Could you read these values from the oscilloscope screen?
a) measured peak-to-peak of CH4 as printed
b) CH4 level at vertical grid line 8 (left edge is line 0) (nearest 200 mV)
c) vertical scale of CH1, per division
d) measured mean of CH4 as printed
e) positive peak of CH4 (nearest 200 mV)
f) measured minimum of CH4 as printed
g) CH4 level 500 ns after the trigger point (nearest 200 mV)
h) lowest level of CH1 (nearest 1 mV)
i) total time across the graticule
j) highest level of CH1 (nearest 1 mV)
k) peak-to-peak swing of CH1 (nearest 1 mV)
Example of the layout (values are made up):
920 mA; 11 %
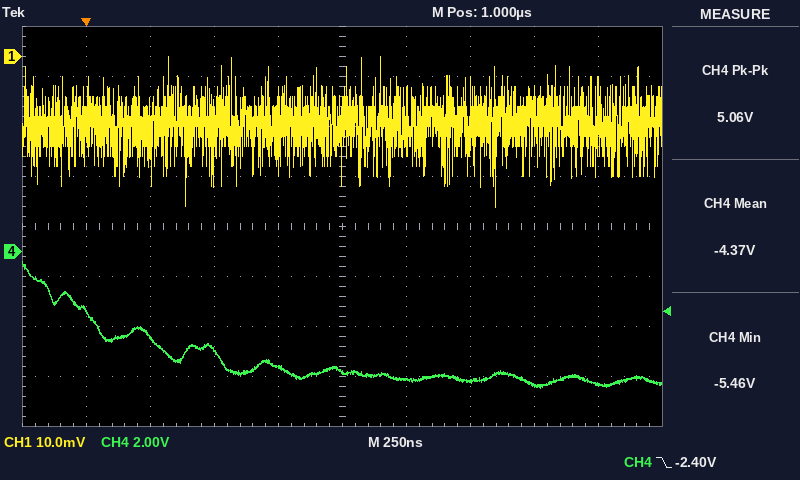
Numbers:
5.06 V; -5.4 V; 10 mV; -4.37 V; -400 mV; -5.46 V; -4.0 V; -30 mV; 2.5 µs; 0 mV; 30 mV
